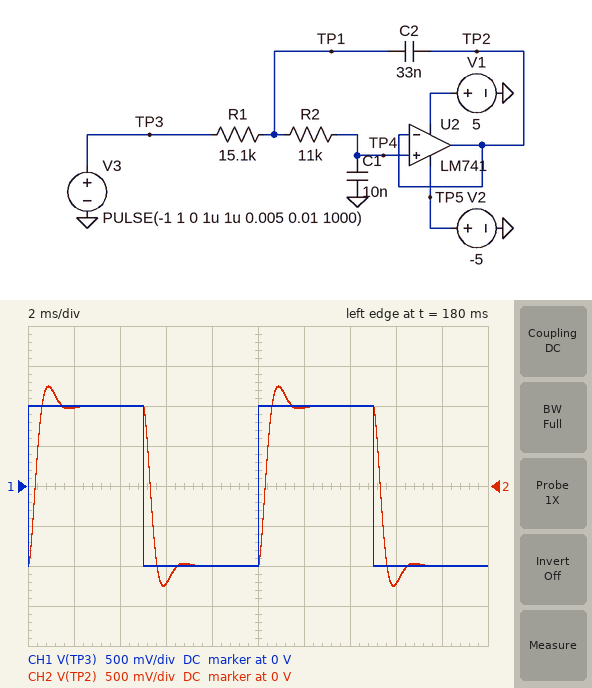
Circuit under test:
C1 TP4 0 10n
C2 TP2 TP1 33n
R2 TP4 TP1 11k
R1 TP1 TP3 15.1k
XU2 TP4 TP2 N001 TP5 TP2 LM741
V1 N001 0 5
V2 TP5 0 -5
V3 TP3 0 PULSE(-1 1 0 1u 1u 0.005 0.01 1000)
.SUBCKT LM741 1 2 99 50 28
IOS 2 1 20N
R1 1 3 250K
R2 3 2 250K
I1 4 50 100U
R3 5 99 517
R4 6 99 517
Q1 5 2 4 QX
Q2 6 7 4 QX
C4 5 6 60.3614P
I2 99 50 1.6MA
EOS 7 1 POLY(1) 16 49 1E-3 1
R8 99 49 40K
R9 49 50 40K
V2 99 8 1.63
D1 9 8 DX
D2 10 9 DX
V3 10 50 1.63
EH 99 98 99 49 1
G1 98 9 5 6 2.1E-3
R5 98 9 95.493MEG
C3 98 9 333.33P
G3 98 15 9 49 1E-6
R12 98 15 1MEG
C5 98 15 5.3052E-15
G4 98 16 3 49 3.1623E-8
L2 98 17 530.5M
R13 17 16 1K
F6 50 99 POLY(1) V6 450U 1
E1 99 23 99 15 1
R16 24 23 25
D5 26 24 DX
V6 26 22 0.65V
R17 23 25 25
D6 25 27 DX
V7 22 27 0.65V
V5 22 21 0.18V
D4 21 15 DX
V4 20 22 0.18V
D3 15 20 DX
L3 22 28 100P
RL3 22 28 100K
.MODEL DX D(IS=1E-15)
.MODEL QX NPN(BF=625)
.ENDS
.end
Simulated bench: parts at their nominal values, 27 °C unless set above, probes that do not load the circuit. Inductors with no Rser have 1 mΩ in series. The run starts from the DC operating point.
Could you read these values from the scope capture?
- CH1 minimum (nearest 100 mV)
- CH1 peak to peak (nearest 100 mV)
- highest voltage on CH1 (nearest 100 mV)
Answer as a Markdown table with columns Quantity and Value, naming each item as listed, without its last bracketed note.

| Quantity | Value |
|---|---|
| CH1 minimum | -1.0 V |
| CH1 peak to peak | 2.0 V |
| highest voltage on CH1 | 1.0 V |
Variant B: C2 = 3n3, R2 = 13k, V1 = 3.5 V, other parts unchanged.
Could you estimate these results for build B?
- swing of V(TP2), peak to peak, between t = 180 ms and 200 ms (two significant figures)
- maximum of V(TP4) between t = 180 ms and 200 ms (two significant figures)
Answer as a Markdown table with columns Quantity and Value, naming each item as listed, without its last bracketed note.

| Quantity | Value |
|---|---|
| swing of V(TP2), peak to peak, between t = 180 ms and 200 ms | 2.0 V |
| maximum of V(TP4) between t = 180 ms and 200 ms | 1.0 V |
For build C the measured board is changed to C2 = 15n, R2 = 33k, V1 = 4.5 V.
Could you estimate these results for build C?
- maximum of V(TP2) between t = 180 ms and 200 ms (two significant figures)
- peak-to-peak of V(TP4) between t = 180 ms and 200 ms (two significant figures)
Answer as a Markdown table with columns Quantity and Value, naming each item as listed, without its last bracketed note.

| Quantity | Value |
|---|---|
| maximum of V(TP2) between t = 180 ms and 200 ms | 1.0 V |
| peak-to-peak of V(TP4) between t = 180 ms and 200 ms | 2.0 V |
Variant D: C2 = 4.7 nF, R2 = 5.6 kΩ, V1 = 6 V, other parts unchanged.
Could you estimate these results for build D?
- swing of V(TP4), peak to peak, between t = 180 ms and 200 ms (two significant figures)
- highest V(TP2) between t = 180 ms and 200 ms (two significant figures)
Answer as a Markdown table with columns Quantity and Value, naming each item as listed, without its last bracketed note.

| Quantity | Value |
|---|---|
| swing of V(TP4), peak to peak, between t = 180 ms and 200 ms | 2.0 V |
| highest V(TP2) between t = 180 ms and 200 ms | 1.0 V |
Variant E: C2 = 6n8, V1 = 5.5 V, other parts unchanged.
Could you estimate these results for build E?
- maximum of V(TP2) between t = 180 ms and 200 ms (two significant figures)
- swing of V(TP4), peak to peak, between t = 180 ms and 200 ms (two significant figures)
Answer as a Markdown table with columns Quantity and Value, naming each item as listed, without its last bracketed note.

| Quantity | Value |
|---|---|
| maximum of V(TP2) between t = 180 ms and 200 ms | 1.0 V |
| swing of V(TP4), peak to peak, between t = 180 ms and 200 ms | 2.0 V |
